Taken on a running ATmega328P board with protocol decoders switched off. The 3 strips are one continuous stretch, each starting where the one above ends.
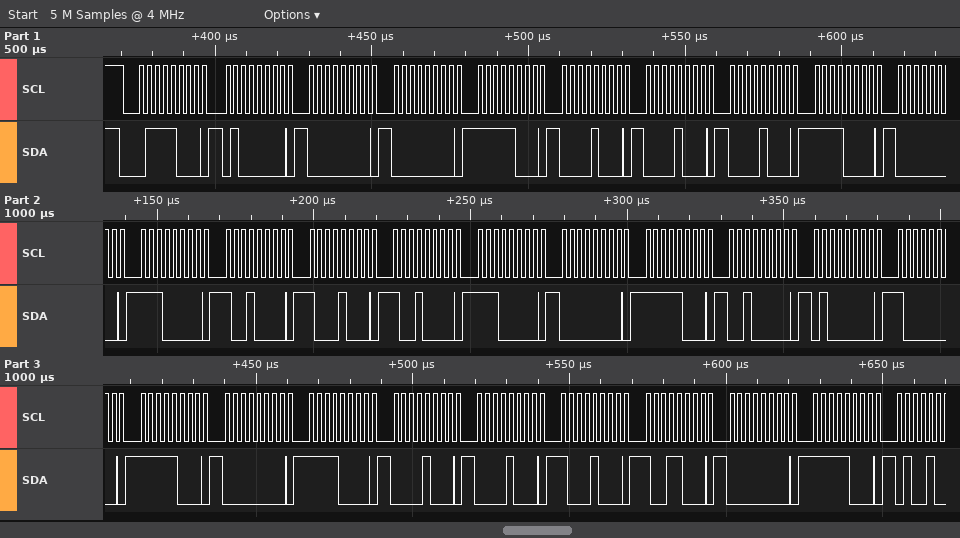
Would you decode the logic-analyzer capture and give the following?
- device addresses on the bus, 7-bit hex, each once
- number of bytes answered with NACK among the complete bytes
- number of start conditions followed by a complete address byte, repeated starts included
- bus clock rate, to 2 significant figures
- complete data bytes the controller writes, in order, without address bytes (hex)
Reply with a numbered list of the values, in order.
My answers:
1. 0x3C
2. 0
3. 1
4. 400 kHz
5. 40 00 00 F8 08 08 08 F0 00 E0 90 88 90 E0 00 F8 20 40 80 F8 00 F0 08 08 88 98 00 F8
